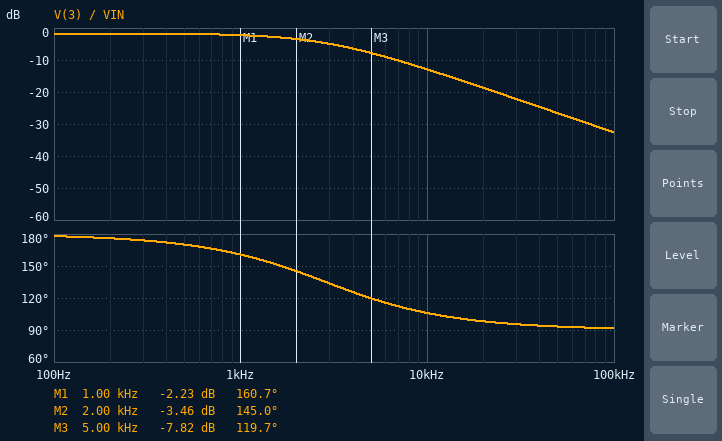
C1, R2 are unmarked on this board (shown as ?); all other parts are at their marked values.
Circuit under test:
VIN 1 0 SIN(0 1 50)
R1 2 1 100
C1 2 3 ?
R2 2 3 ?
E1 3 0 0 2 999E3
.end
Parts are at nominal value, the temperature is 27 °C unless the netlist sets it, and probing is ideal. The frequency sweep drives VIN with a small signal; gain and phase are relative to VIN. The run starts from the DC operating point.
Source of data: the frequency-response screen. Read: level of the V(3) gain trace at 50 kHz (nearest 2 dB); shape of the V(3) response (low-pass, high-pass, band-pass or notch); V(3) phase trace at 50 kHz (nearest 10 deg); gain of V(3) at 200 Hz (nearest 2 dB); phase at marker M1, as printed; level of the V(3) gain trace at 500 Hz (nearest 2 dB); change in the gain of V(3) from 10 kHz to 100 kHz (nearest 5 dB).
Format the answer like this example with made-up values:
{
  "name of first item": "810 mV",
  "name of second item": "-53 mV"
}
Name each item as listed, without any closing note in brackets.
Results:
{
  "level of the V(3) gain trace at 50 kHz": "-26 dB",
  "shape of the V(3) response": "low-pass",
  "V(3) phase trace at 50 kHz": "90 deg",
  "gain of V(3) at 200 Hz": "-2 dB",
  "phase at marker M1, as printed": "160.7 deg",
  "level of the V(3) gain trace at 500 Hz": "-2 dB",
  "change in the gain of V(3) from 10 kHz to 100 kHz": "-20 dB"
}
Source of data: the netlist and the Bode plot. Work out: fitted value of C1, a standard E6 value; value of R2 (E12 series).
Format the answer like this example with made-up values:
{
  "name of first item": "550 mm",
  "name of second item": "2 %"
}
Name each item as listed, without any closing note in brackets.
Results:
{
  "fitted value of C1, a standard E6 value": "680 nF",
  "value of R2": "82 Ω"
}
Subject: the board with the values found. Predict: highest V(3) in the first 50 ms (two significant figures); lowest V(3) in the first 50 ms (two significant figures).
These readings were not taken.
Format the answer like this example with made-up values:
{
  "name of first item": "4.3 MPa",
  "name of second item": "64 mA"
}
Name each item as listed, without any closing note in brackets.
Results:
{
  "highest V(3) in the first 50 ms": "820 mV",
  "lowest V(3) in the first 50 ms": "-820 mV"
}
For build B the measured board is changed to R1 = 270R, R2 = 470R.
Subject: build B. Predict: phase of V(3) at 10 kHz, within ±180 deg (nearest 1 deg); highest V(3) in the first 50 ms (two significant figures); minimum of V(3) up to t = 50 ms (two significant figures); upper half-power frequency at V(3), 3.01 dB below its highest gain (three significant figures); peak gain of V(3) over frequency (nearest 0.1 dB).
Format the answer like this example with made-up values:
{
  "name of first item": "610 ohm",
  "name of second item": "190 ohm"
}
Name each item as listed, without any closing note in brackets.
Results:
{
  "phase of V(3) at 10 kHz, within ±180 deg": "93 deg",
  "highest V(3) in the first 50 ms": "1.7 V",
  "minimum of V(3) up to t = 50 ms": "-1.7 V",
  "upper half-power frequency at V(3), 3.01 dB below its highest gain": "498 Hz",
  "peak gain of V(3) over frequency": "4.8 dB"
}
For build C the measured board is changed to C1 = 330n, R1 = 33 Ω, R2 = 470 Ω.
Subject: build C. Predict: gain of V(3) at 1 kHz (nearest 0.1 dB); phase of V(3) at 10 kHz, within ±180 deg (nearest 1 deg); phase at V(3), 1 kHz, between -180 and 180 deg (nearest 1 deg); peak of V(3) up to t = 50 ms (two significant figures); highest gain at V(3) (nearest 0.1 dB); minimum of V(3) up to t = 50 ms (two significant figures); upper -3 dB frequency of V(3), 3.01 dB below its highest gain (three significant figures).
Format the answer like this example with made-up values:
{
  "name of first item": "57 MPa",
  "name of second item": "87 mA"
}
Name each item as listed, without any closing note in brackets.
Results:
{
  "gain of V(3) at 1 kHz": "20.2 dB",
  "phase of V(3) at 10 kHz, within ±180 deg": "96 deg",
  "phase at V(3), 1 kHz, between -180 and 180 deg": "136 deg",
  "peak of V(3) up to t = 50 ms": "14 V",
  "highest gain at V(3)": "23.1 dB",
  "minimum of V(3) up to t = 50 ms": "-14 V",
  "upper -3 dB frequency of V(3), 3.01 dB below its highest gain": "1.03 kHz"
}
